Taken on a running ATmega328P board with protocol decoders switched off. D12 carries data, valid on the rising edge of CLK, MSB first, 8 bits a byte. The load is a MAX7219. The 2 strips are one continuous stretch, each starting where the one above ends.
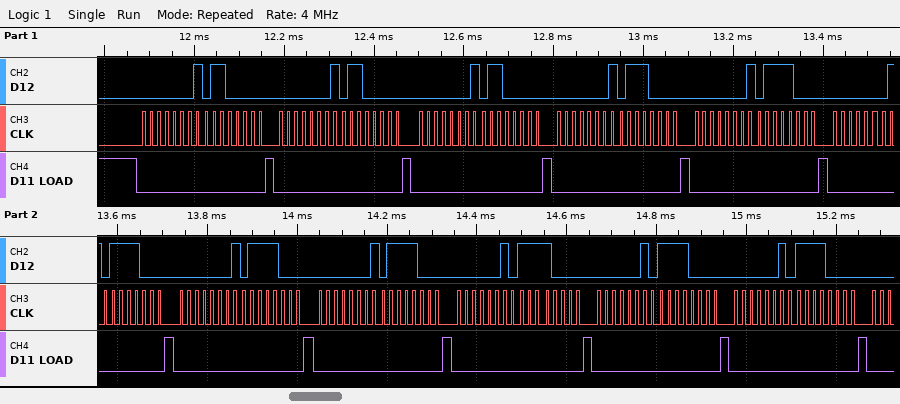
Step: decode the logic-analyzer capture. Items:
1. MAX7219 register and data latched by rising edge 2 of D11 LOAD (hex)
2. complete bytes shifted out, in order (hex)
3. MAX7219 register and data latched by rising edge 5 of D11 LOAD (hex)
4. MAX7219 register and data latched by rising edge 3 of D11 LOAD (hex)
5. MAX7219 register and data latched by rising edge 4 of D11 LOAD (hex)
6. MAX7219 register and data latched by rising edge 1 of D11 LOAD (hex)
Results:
register 0x1, data 0x60
0x01 0x60 0x01 0x60 0x01 0x60 0x01 0x70 0x01 0x78 0x01 0x78 0x01 0x78 0x01 0x78 0x02 0xF0 0x02 0xF0 0x02 0xF0
register 0x1, data 0x78
register 0x1, data 0x60
register 0x1, data 0x70
register 0x1, data 0x60
